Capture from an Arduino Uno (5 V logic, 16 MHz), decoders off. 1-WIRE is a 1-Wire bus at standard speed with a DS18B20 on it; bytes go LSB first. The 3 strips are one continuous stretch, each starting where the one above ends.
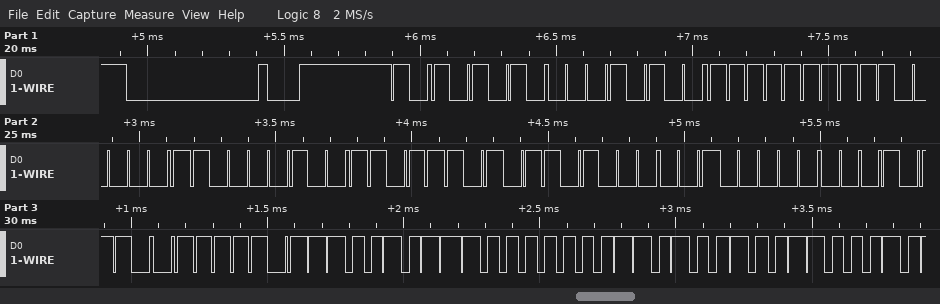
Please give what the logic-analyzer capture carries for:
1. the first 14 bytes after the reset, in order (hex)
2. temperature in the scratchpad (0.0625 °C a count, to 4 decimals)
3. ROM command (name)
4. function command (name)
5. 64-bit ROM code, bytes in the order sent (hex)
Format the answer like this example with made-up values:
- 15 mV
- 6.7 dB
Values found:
- 55 28 FF 83 21 BB 16 04 68 BE D3 01 4B 46
- 29.1875 °C
- Match ROM
- Read Scratchpad
- 28 FF 83 21 BB 16 04 68
